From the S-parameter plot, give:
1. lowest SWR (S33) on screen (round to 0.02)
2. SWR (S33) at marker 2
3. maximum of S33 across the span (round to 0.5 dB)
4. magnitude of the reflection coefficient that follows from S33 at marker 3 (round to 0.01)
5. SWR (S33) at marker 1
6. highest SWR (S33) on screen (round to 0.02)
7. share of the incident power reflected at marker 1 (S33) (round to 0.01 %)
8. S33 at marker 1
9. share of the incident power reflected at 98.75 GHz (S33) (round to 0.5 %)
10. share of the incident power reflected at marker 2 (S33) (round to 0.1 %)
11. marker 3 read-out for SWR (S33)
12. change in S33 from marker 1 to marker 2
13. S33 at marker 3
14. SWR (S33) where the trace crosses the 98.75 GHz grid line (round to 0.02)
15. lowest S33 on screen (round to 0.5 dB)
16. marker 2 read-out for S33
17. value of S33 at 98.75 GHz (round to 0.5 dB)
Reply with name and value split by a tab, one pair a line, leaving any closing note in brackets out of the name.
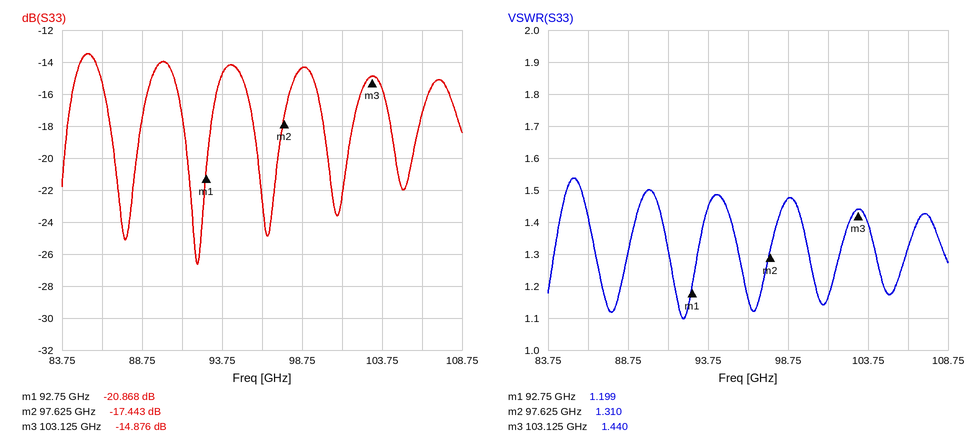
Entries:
lowest SWR (S33) on screen	1.10
SWR (S33) at marker 2	1.310
maximum of S33 across the span	-13.5 dB
magnitude of the reflection coefficient that follows from S33 at marker 3	0.18
SWR (S33) at marker 1	1.199
highest SWR (S33) on screen	1.54
share of the incident power reflected at marker 1 (S33)	0.82 %
S33 at marker 1	-20.868 dB
share of the incident power reflected at 98.75 GHz (S33)	3.5 %
share of the incident power reflected at marker 2 (S33)	1.8 %
marker 3 read-out for SWR	1.440
change in S33 from marker 1 to marker 2	3.425 dB
S33 at marker 3	-14.876 dB
SWR (S33) where the trace crosses the 98.75 GHz grid line	1.48
lowest S33 on screen	-26.5 dB
marker 2 read-out for S33	-17.443 dB
value of S33 at 98.75 GHz	-14.5 dB
